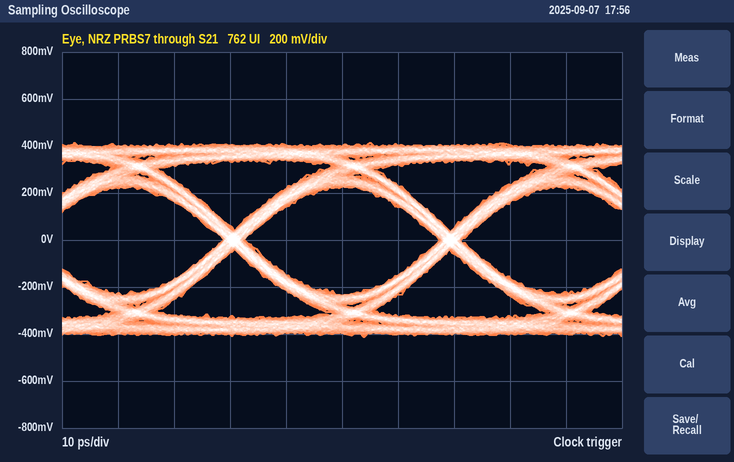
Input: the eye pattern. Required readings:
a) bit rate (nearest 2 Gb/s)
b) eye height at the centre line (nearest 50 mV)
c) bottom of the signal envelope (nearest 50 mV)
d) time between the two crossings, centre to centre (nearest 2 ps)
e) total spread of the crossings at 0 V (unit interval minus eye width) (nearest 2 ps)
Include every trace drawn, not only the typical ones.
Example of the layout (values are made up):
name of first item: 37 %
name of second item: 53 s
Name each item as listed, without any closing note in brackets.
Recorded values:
bit rate: 26 Gb/s
eye height at the centre line: 450 mV
bottom of the signal envelope: -400 mV
time between the two crossings, centre to centre: 38 ps
total spread of the crossings at 0 V (unit interval minus eye width): 4 ps
